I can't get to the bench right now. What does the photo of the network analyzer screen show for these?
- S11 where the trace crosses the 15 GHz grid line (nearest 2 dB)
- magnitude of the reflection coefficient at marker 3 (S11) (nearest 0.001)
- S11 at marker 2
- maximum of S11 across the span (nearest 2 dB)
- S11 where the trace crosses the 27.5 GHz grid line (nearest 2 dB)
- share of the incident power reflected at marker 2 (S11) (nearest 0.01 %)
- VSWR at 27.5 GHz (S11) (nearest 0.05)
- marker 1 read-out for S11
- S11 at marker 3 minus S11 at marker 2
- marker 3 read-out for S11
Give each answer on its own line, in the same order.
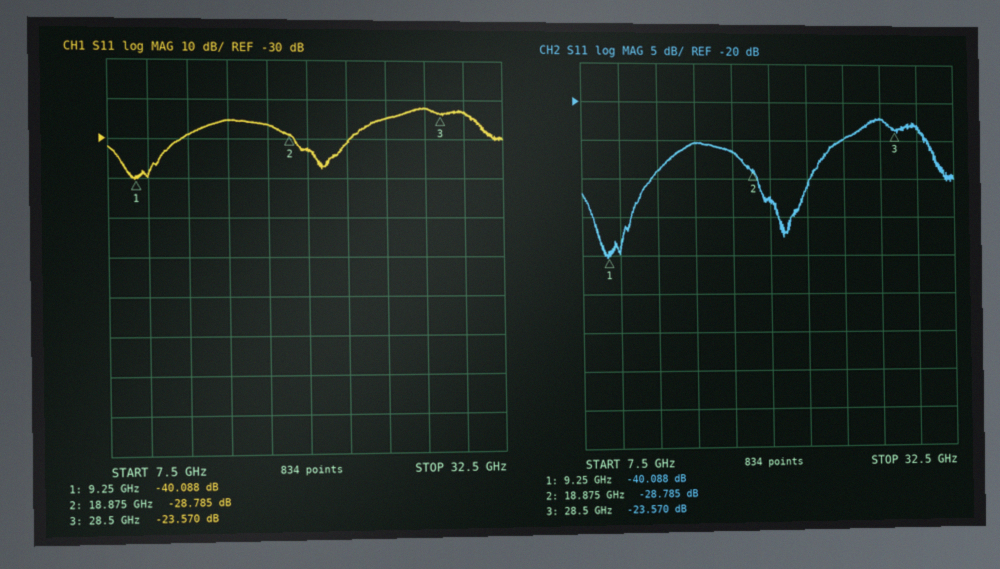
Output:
-26 dB
0.066
-28.785 dB
-22 dB
-22 dB
0.13 %
1.15
-40.088 dB
5.215 dB
-23.570 dB
